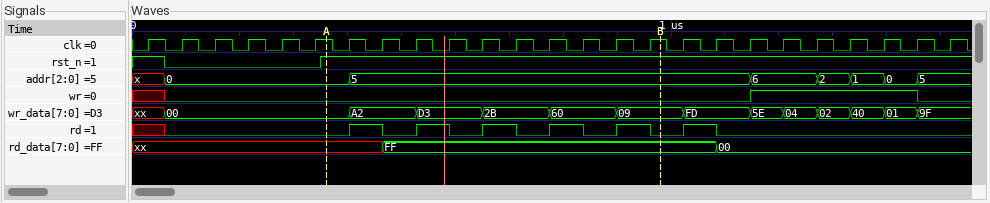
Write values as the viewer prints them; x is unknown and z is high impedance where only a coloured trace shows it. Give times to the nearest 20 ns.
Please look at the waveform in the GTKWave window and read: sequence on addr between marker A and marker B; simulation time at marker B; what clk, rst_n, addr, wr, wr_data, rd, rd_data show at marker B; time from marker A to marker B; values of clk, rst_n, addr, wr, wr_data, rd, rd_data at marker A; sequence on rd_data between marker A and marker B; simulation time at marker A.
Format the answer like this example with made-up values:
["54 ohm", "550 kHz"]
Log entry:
["0, 5", "980 ns", "clk=1, rst_n=1, addr=5, wr=0, wr_data=09, rd=0, rd_data=FF", "620 ns", "clk=1, rst_n=1, addr=0, wr=0, wr_data=00, rd=0, rd_data=xx", "xx, FF", "360 ns"]
